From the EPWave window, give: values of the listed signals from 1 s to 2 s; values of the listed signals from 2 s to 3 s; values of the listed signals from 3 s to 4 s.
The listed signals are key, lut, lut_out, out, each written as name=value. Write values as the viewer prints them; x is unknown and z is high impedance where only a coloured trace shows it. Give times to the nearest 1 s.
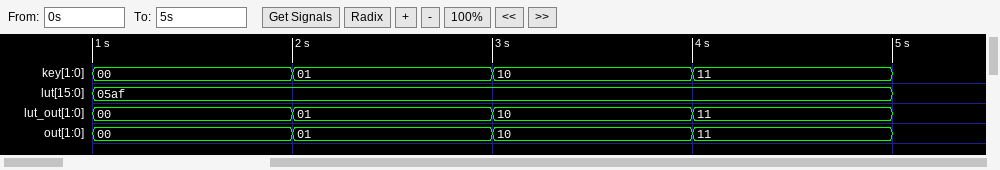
key=00, lut=05af, lut_out=00, out=00
key=01, lut=05af, lut_out=01, out=01
key=10, lut=05af, lut_out=10, out=10
